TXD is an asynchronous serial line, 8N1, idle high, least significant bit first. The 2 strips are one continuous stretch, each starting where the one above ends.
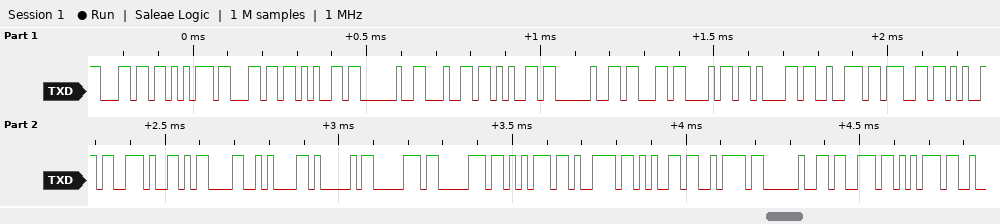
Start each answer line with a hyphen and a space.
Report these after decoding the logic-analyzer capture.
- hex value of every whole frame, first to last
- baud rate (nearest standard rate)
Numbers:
- 6C 75 6C 65 20 64 65 20 63 68 61 72 67 65 2E 0D 0A 41 70 70 75 79 65 7A 20 73 75
- 57600 baud
